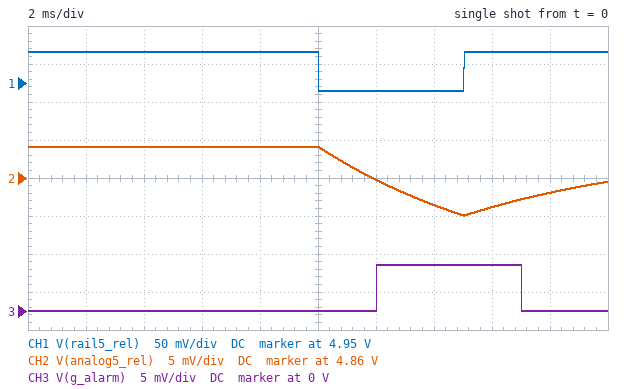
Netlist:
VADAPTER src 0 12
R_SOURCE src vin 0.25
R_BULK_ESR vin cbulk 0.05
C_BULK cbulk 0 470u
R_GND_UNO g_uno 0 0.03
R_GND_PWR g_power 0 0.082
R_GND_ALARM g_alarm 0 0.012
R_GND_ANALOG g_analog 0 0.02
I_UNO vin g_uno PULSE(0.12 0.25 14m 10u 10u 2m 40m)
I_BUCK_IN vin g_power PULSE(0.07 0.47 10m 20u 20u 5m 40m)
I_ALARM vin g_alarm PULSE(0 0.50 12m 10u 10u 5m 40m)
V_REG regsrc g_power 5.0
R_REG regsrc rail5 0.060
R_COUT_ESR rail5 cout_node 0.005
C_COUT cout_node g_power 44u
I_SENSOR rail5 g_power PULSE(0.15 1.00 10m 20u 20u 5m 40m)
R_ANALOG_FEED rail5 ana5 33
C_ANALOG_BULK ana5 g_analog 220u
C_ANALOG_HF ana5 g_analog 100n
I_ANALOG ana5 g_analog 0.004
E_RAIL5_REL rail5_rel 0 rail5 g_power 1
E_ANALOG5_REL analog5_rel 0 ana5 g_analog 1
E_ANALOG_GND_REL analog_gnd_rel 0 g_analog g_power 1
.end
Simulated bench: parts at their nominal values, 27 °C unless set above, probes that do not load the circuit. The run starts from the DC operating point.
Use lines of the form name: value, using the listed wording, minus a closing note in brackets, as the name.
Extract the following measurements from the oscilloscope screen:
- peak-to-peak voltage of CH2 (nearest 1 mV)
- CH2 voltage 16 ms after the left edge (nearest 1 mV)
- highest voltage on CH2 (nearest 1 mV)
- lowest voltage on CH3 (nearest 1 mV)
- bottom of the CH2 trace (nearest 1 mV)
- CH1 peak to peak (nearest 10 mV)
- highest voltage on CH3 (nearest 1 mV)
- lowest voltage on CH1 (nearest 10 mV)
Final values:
peak-to-peak voltage of CH2: 9 mV
CH2 voltage 16 ms after the left edge: 4.856 V
highest voltage on CH2: 4.864 V
lowest voltage on CH3: 0 V
bottom of the CH2 trace: 4.855 V
CH1 peak to peak: 50 mV
highest voltage on CH3: 6 mV
lowest voltage on CH1: 4.94 V
